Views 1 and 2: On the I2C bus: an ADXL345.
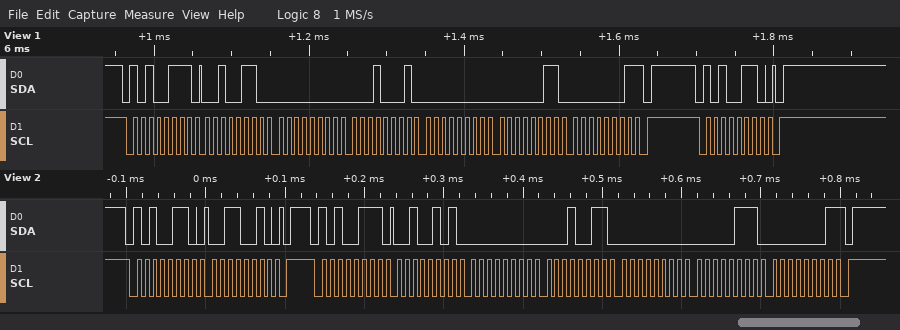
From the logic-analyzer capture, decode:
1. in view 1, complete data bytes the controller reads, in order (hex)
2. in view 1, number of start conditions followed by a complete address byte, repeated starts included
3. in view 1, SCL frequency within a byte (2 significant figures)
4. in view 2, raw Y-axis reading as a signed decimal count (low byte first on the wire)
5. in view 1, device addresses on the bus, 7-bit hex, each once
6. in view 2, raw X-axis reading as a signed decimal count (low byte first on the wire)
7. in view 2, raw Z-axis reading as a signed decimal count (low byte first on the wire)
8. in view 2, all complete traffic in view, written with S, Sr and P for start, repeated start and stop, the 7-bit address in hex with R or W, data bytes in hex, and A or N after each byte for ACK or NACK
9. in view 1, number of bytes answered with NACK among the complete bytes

26 00 11 00 03 01
2
100 kHz
19
0x53
37
263
S 53W A 32 A P S 53R A 25 A 00 A 13 A 00 A 07 A 01 N P
1
